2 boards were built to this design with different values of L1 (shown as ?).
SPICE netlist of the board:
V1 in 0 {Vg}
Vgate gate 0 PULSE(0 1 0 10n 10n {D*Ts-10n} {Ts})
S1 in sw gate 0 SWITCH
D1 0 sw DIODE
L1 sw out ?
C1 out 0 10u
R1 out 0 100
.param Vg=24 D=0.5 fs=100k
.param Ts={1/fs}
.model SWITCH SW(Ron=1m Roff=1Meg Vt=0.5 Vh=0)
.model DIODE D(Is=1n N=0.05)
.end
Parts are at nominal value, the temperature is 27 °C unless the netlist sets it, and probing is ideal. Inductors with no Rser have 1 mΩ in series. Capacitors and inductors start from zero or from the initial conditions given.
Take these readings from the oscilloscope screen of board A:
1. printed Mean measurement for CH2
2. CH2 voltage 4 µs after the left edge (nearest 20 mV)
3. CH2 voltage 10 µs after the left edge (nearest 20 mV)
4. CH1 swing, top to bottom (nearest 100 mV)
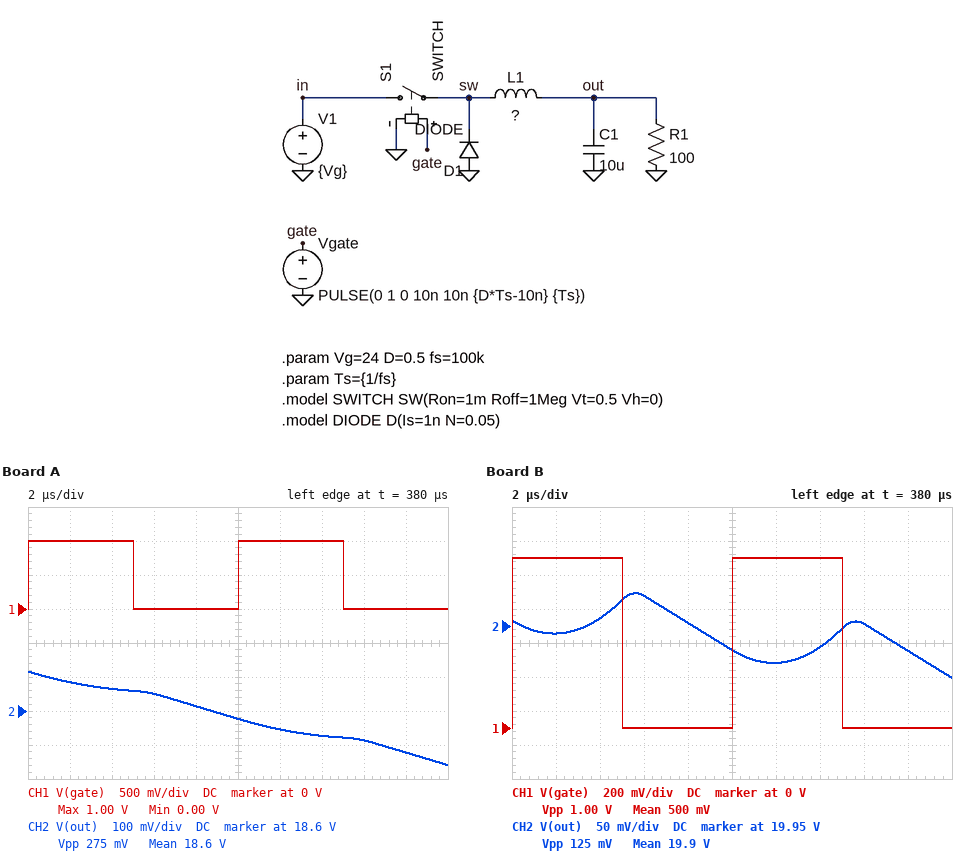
18.6 V
18.66 V
18.58 V
1.0 V
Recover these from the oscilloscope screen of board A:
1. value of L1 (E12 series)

180 µH
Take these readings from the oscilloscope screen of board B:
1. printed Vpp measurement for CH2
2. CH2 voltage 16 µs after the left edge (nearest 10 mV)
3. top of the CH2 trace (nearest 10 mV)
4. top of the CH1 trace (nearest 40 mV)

125 mV
19.95 V
20.00 V
1.00 V
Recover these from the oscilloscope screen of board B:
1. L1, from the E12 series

39 µH
